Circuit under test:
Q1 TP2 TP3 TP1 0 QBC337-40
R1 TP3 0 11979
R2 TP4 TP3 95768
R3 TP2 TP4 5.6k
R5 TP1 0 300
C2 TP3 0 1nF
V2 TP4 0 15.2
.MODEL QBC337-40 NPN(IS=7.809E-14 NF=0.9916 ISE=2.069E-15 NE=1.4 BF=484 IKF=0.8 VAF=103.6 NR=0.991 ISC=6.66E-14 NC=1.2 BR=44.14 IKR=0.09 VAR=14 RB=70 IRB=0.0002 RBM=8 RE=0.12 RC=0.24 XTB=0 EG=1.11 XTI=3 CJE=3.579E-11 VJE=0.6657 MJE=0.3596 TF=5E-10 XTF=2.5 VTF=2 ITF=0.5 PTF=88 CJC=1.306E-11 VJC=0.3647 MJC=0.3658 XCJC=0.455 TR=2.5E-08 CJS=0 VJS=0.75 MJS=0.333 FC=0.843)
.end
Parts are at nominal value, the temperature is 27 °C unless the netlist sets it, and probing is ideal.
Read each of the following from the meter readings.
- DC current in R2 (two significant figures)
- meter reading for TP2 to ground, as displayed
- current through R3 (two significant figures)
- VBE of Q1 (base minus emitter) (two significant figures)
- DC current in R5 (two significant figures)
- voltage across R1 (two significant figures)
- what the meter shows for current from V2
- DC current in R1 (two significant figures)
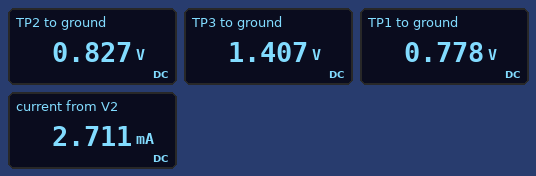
140 µA
0.827 V
2.6 mA
630 mV
2.6 mA
1.4 V
2.711 mA
120 µA
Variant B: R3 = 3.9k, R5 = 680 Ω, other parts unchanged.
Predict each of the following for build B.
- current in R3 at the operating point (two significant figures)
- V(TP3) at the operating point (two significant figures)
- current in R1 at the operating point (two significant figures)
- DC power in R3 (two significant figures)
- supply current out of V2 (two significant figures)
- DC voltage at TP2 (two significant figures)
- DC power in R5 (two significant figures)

1.5 mA
1.7 V
140 µA
9.2 mW
1.7 mA
9.2 V
1.6 mW
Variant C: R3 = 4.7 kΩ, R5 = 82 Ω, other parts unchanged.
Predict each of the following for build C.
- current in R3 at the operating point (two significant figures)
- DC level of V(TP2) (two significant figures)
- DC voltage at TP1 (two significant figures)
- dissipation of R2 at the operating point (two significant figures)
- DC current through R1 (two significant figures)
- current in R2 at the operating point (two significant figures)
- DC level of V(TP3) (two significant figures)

3.2 mA
300 mV
270 mV
2.1 mW
76 µA
150 µA
910 mV
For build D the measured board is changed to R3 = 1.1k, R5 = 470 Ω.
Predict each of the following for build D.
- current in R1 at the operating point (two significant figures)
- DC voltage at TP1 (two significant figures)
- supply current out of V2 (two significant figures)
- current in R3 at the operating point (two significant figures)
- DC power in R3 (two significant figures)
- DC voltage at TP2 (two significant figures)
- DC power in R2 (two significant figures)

140 µA
1.0 V
2.3 mA
2.2 mA
5.2 mW
13 V
1.9 mW
